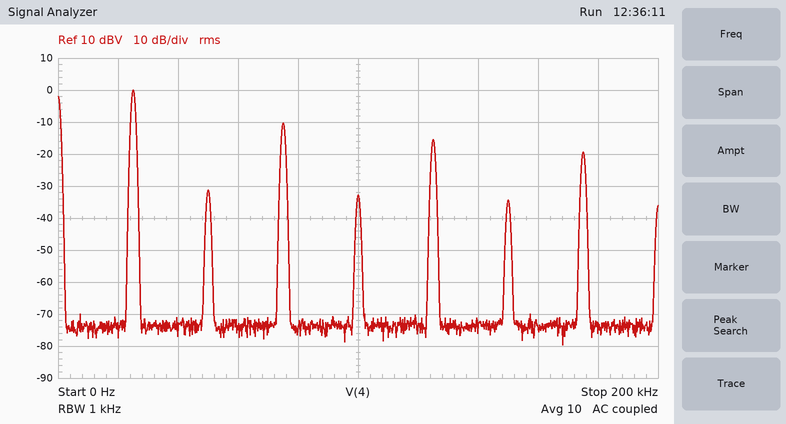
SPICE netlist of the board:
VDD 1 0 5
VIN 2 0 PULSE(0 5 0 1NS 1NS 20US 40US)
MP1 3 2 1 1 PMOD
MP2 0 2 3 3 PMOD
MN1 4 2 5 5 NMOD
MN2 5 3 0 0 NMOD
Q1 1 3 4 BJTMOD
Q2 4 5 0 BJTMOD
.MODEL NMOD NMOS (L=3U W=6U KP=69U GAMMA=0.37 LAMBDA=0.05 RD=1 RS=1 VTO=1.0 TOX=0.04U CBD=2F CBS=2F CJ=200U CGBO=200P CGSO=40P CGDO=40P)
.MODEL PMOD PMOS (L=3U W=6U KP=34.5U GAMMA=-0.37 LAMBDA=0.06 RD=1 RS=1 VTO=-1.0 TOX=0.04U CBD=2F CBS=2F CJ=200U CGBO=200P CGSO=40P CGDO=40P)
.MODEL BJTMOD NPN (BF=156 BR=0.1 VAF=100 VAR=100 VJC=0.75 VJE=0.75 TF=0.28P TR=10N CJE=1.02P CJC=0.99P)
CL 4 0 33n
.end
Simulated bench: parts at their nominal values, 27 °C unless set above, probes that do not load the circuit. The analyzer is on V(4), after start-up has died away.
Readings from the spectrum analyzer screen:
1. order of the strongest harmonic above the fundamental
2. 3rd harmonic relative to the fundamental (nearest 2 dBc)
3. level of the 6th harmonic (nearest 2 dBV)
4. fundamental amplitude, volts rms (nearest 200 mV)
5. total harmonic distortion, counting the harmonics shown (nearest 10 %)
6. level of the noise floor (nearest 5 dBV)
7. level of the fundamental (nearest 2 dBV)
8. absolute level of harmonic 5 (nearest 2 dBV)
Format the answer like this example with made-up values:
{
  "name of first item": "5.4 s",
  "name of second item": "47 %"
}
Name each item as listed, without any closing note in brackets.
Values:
{
  "order of the strongest harmonic above the fundamental": "3",
  "3rd harmonic relative to the fundamental": "-10 dBc",
  "level of the 6th harmonic": "-34 dBV",
  "fundamental amplitude, volts rms": "1.0 V",
  "total harmonic distortion, counting the harmonics shown": "40 %",
  "level of the noise floor": "-75 dBV",
  "level of the fundamental": "0 dBV",
  "absolute level of harmonic 5": "-16 dBV"
}
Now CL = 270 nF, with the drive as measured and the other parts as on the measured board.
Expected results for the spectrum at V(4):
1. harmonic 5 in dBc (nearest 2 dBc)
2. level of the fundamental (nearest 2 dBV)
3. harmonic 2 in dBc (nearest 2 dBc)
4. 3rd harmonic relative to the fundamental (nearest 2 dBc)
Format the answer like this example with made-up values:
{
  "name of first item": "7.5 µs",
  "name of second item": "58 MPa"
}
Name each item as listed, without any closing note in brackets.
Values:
{
  "harmonic 5 in dBc": "-26 dBc",
  "level of the fundamental": "-4 dBV",
  "harmonic 2 in dBc": "-22 dBc",
  "3rd harmonic relative to the fundamental": "-16 dBc"
}
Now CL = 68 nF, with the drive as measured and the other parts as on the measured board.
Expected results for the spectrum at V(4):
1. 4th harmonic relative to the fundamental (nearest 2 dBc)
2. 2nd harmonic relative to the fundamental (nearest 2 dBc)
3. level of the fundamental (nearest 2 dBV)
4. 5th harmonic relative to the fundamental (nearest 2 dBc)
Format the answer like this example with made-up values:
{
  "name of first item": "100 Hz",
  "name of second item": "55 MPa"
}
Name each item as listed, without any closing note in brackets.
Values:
{
  "4th harmonic relative to the fundamental": "-30 dBc",
  "2nd harmonic relative to the fundamental": "-26 dBc",
  "level of the fundamental": "0 dBV",
  "5th harmonic relative to the fundamental": "-18 dBc"
}
